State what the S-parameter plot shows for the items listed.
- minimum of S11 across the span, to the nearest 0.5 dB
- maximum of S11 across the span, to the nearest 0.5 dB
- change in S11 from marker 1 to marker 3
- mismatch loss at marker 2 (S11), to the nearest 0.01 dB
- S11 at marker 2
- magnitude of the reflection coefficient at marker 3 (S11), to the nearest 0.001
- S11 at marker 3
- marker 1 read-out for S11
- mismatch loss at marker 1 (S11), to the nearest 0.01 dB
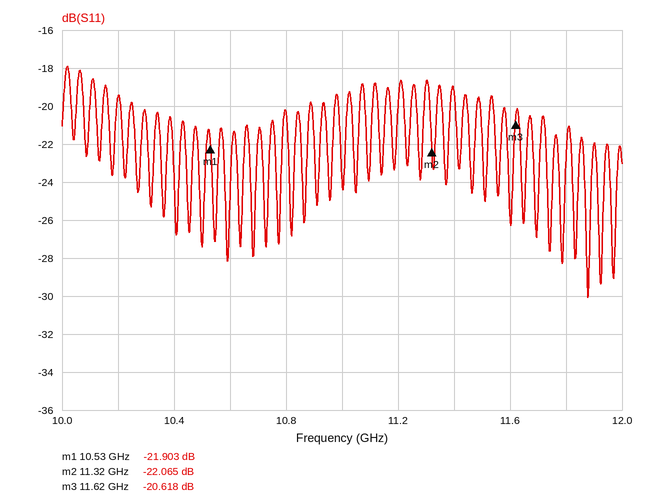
-30.0 dB
-18.0 dB
1.285 dB
0.03 dB
-22.065 dB
0.093
-20.618 dB
-21.903 dB
0.03 dB
